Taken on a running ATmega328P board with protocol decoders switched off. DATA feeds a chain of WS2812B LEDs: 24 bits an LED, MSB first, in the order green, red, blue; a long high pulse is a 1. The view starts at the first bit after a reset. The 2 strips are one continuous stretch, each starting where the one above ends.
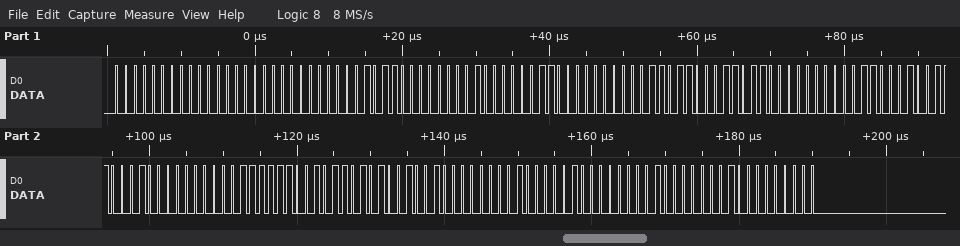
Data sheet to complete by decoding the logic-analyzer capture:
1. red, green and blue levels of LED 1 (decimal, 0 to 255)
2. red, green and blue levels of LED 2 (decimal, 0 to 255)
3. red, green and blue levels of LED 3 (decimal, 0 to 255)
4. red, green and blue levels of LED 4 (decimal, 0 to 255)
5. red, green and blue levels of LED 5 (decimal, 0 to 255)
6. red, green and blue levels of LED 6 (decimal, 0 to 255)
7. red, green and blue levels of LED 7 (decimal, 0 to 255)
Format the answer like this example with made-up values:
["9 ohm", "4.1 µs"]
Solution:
["0, 0, 0", "1, 22, 3", "54, 0, 54", "98, 0, 98", "126, 0, 90", "1, 146, 4", "2, 2, 0"]
